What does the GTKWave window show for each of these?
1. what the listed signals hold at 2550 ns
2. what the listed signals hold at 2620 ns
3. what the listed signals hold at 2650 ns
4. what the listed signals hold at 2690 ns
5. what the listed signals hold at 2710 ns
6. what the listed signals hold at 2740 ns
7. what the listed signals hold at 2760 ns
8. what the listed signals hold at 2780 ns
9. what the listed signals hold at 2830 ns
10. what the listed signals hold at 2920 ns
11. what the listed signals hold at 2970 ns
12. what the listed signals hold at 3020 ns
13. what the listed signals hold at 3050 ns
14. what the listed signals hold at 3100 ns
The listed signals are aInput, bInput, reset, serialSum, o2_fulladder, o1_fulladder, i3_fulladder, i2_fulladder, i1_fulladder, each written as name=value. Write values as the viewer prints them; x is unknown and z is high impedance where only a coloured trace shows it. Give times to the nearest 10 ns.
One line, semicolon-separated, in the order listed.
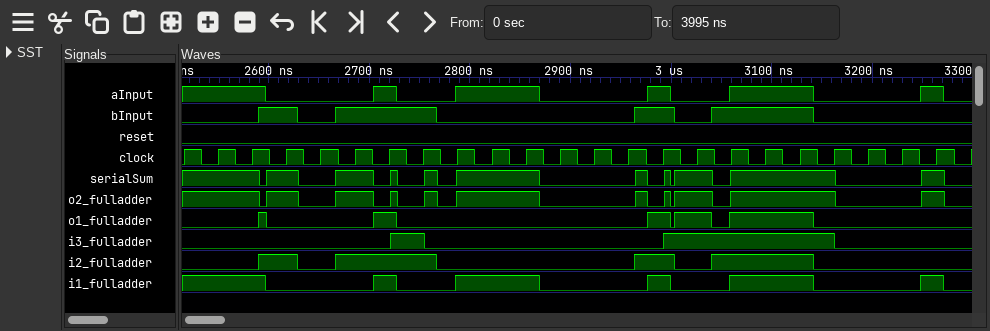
aInput=1, bInput=0, reset=0, serialSum=1, o2_fulladder=1, o1_fulladder=0, i3_fulladder=0, i2_fulladder=0, i1_fulladder=1; aInput=0, bInput=1, reset=0, serialSum=1, o2_fulladder=1, o1_fulladder=0, i3_fulladder=0, i2_fulladder=1, i1_fulladder=0; aInput=0, bInput=0, reset=0, serialSum=0, o2_fulladder=0, o1_fulladder=0, i3_fulladder=0, i2_fulladder=0, i1_fulladder=0; aInput=0, bInput=1, reset=0, serialSum=1, o2_fulladder=1, o1_fulladder=0, i3_fulladder=0, i2_fulladder=1, i1_fulladder=0; aInput=1, bInput=1, reset=0, serialSum=0, o2_fulladder=0, o1_fulladder=1, i3_fulladder=0, i2_fulladder=1, i1_fulladder=1; aInput=0, bInput=1, reset=0, serialSum=0, o2_fulladder=0, o1_fulladder=0, i3_fulladder=1, i2_fulladder=1, i1_fulladder=0; aInput=0, bInput=1, reset=0, serialSum=1, o2_fulladder=1, o1_fulladder=0, i3_fulladder=0, i2_fulladder=1, i1_fulladder=0; aInput=0, bInput=0, reset=0, serialSum=0, o2_fulladder=0, o1_fulladder=0, i3_fulladder=0, i2_fulladder=0, i1_fulladder=0; aInput=1, bInput=0, reset=0, serialSum=1, o2_fulladder=1, o1_fulladder=0, i3_fulladder=0, i2_fulladder=0, i1_fulladder=1; aInput=0, bInput=0, reset=0, serialSum=0, o2_fulladder=0, o1_fulladder=0, i3_fulladder=0, i2_fulladder=0, i1_fulladder=0; aInput=0, bInput=1, reset=0, serialSum=1, o2_fulladder=1, o1_fulladder=0, i3_fulladder=0, i2_fulladder=1, i1_fulladder=0; aInput=0, bInput=0, reset=0, serialSum=1, o2_fulladder=1, o1_fulladder=1, i3_fulladder=1, i2_fulladder=0, i1_fulladder=0; aInput=0, bInput=1, reset=0, serialSum=0, o2_fulladder=0, o1_fulladder=0, i3_fulladder=1, i2_fulladder=1, i1_fulladder=0; aInput=1, bInput=1, reset=0, serialSum=1, o2_fulladder=1, o1_fulladder=1, i3_fulladder=1, i2_fulladder=1, i1_fulladder=1
